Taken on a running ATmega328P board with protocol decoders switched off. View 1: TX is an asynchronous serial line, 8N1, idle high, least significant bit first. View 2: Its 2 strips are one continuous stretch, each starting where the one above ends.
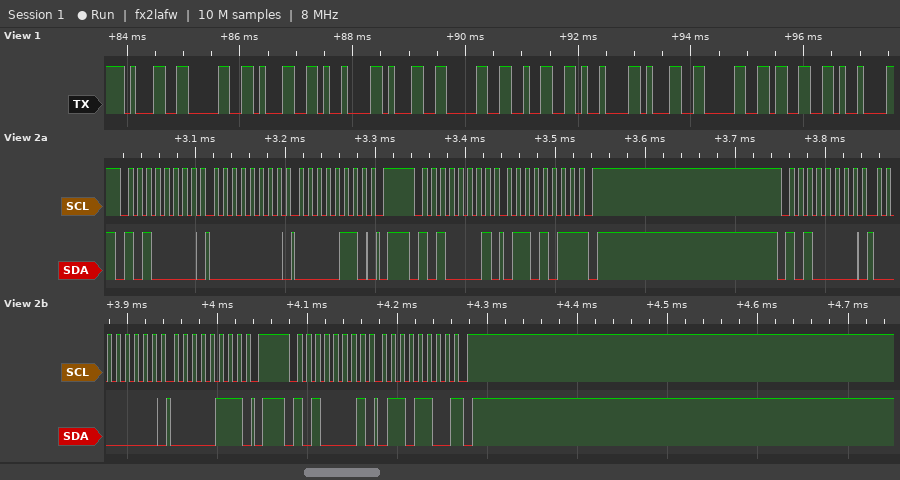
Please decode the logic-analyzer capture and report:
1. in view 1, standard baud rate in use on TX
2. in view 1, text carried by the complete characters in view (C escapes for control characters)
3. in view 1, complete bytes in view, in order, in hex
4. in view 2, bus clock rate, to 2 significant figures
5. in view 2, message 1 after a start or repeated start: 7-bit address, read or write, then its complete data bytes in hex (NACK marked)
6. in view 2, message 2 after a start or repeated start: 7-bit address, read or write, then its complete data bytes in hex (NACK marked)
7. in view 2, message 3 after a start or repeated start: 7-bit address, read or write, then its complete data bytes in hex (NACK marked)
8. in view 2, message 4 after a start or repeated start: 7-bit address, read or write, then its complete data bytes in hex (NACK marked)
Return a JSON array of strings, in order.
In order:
["9600 baud", "\"101\\t102\\t103\\t\"", "0x31 0x30 0x31 0x09 0x31 0x30 0x32 0x09 0x31 0x30 0x33 0x09", "100 kHz", "0x50 write: 00 06", "0x50 read: 6B NACK", "0x50 write: 00 07", "0x50 read: 6C NACK"]
